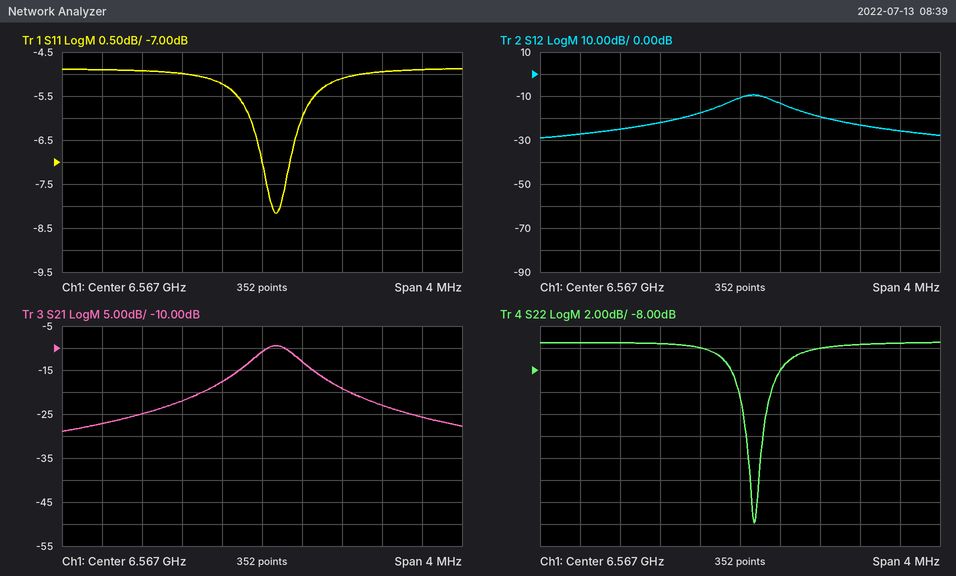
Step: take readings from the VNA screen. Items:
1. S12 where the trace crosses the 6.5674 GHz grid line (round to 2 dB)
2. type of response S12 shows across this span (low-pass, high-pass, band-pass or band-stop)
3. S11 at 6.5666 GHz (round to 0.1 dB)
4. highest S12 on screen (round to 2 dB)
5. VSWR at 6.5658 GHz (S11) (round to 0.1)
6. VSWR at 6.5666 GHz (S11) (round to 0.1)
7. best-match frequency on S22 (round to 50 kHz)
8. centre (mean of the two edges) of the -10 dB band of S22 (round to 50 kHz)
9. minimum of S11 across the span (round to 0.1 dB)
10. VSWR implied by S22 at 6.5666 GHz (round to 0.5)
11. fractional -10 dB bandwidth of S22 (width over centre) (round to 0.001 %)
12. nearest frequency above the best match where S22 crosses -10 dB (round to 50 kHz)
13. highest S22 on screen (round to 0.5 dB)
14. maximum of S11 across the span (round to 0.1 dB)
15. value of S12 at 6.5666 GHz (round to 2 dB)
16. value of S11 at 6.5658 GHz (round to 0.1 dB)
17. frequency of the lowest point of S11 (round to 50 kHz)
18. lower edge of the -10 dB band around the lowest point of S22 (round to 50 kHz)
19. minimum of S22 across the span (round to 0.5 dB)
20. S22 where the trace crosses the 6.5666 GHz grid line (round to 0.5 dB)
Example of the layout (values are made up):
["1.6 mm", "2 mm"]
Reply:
["-14 dB", "band-pass", "-5.2 dB", "-10 dB", "3.6", "3.4", "6.56715 GHz", "6.56715 GHz", "-8.2 dB", "3.0", "0.005 %", "6.56730 GHz", "-5.5 dB", "-4.9 dB", "-18 dB", "-4.9 dB", "6.56715 GHz", "6.56700 GHz", "-22.0 dB", "-6.0 dB"]
